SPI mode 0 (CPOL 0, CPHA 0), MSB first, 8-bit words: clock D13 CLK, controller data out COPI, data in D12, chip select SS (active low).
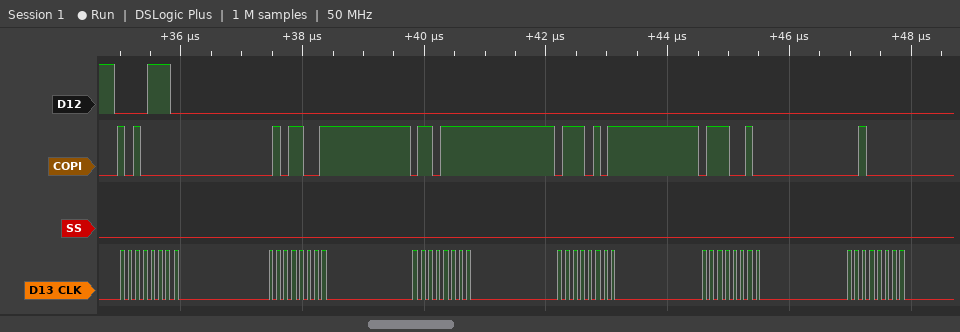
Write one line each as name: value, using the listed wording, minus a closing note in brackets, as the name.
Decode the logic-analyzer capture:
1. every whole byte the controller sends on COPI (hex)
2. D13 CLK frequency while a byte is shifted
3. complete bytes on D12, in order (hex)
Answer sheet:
every whole byte the controller sends on COPI: A0 59 6F 75 72 20
D13 CLK frequency while a byte is shifted: 8 MHz
complete bytes on D12, in order: 0E 00 00 00 00 00
